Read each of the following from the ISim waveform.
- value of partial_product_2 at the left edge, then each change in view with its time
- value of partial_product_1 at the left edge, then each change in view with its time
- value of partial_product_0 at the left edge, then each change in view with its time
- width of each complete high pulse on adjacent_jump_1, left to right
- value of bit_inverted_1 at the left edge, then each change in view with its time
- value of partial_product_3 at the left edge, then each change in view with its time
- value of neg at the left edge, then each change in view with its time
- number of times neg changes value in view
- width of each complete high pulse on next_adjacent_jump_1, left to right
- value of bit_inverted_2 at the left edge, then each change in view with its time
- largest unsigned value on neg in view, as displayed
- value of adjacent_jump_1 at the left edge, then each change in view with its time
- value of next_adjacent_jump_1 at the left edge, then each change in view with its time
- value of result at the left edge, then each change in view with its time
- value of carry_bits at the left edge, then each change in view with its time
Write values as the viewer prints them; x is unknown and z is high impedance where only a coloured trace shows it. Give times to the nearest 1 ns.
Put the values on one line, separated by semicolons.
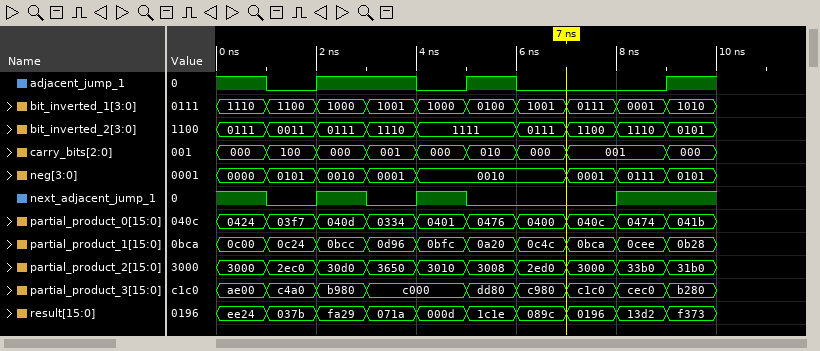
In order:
3000, 2ec0 at 1 ns, 30d0 at 2 ns, 3650 at 3 ns, 3010 at 4 ns, 3008 at 5 ns, 2ed0 at 6 ns, 3000 at 7 ns, 33b0 at 8 ns, 31b0 at 9 ns; 0c00, 0c24 at 1 ns, 0bcc at 2 ns, 0d96 at 3 ns, 0bfc at 4 ns, 0a20 at 5 ns, 0c4c at 6 ns, 0bca at 7 ns, 0cee at 8 ns, 0b28 at 9 ns; 0424, 03f7 at 1 ns, 040d at 2 ns, 0334 at 3 ns, 0401 at 4 ns, 0476 at 5 ns, 0400 at 6 ns, 040c at 7 ns, 0474 at 8 ns, 041b at 9 ns; 2 ns, 1 ns; 1110, 1100 at 1 ns, 1000 at 2 ns, 1001 at 3 ns, 1000 at 4 ns, 0100 at 5 ns, 1001 at 6 ns, 0111 at 7 ns, 0001 at 8 ns, 1010 at 9 ns; ae00, c4a0 at 1 ns, b980 at 2 ns, c000 at 3 ns, dd80 at 5 ns, c980 at 6 ns, c1c0 at 7 ns, cec0 at 8 ns, b280 at 9 ns; 0000, 0101 at 1 ns, 0010 at 2 ns, 0001 at 3 ns, 0010 at 4 ns, 0001 at 7 ns, 0111 at 8 ns, 0101 at 9 ns; 7; 1 ns, 1 ns; 0111, 0011 at 1 ns, 0111 at 2 ns, 1110 at 3 ns, 1111 at 4 ns, 0111 at 6 ns, 1100 at 7 ns, 1110 at 8 ns, 0101 at 9 ns; 0111; 1, 0 at 1 ns, 1 at 2 ns, 0 at 4 ns, 1 at 5 ns, 0 at 6 ns, 1 at 9 ns; 1, 0 at 1 ns, 1 at 2 ns, 0 at 3 ns, 1 at 4 ns, 0 at 5 ns, 1 at 8 ns; ee24, 037b at 1 ns, fa29 at 2 ns, 071a at 3 ns, 000d at 4 ns, 1c1e at 5 ns, 089c at 6 ns, 0196 at 7 ns, 13d2 at 8 ns, f373 at 9 ns; 000, 100 at 1 ns, 000 at 2 ns, 001 at 3 ns, 000 at 4 ns, 010 at 5 ns, 000 at 6 ns, 001 at 7 ns, 000 at 9 ns
